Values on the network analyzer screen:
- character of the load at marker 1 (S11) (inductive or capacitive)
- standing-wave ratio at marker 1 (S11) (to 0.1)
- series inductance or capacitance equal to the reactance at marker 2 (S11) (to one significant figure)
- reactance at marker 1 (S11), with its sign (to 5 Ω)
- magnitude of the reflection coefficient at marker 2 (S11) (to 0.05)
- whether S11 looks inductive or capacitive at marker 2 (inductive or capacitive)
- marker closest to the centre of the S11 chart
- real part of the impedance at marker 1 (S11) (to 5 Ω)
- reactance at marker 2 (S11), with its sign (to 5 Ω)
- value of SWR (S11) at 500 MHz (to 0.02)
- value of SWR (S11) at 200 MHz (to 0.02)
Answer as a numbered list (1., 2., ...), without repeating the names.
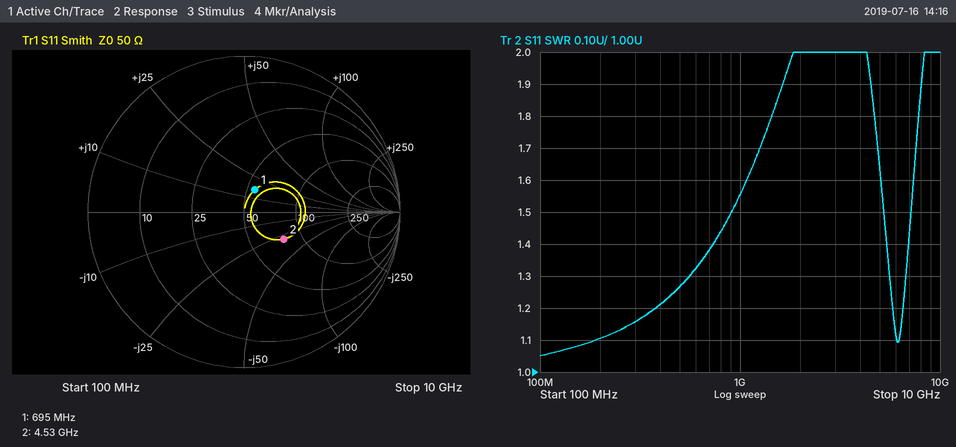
1. inductive
2. 1.4
3. 1 pF
4. +15 Ω
5. 0.30
6. capacitive
7. marker 1
8. 55 Ω
9. -30 Ω
10. 1.26
11. 1.10
